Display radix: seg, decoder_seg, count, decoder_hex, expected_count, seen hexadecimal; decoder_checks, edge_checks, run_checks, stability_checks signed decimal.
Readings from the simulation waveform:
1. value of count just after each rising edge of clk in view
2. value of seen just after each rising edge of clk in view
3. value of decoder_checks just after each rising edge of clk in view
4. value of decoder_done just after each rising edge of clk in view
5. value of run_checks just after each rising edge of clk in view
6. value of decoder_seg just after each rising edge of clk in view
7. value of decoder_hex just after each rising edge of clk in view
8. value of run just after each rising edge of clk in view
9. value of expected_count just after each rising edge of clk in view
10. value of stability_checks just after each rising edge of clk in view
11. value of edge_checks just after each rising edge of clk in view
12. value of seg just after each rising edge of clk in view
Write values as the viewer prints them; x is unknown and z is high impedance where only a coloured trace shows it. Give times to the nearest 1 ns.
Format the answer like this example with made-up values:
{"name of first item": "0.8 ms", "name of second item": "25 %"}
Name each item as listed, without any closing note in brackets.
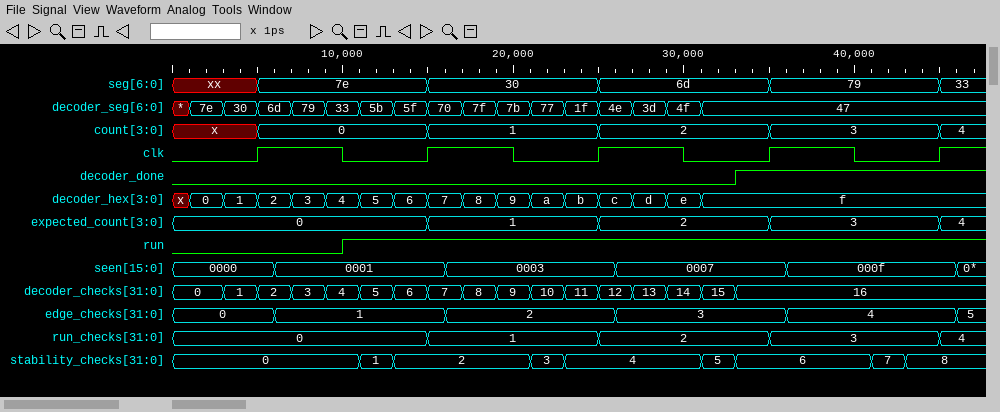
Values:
{"value of count just after each rising edge of clk in view": "0, 1, 2, 3, 4", "value of seen just after each rising edge of clk in view": "0000, 0001, 0003, 0007, 000f", "value of decoder_checks just after each rising edge of clk in view": "2, 7, 12, 16, 16", "value of decoder_done just after each rising edge of clk in view": "0 0 0 1 1", "value of run_checks just after each rising edge of clk in view": "0, 1, 2, 3, 4", "value of decoder_seg just after each rising edge of clk in view": "6d, 70, 4e, 47, 47", "value of decoder_hex just after each rising edge of clk in view": "2, 7, c, f, f", "value of run just after each rising edge of clk in view": "0 1 1 1 1", "value of expected_count just after each rising edge of clk in view": "0, 1, 2, 3, 4", "value of stability_checks just after each rising edge of clk in view": "0, 2, 4, 6, 8", "value of edge_checks just after each rising edge of clk in view": "0, 1, 2, 3, 4", "value of seg just after each rising edge of clk in view": "7e, 30, 6d, 79, 33"}
